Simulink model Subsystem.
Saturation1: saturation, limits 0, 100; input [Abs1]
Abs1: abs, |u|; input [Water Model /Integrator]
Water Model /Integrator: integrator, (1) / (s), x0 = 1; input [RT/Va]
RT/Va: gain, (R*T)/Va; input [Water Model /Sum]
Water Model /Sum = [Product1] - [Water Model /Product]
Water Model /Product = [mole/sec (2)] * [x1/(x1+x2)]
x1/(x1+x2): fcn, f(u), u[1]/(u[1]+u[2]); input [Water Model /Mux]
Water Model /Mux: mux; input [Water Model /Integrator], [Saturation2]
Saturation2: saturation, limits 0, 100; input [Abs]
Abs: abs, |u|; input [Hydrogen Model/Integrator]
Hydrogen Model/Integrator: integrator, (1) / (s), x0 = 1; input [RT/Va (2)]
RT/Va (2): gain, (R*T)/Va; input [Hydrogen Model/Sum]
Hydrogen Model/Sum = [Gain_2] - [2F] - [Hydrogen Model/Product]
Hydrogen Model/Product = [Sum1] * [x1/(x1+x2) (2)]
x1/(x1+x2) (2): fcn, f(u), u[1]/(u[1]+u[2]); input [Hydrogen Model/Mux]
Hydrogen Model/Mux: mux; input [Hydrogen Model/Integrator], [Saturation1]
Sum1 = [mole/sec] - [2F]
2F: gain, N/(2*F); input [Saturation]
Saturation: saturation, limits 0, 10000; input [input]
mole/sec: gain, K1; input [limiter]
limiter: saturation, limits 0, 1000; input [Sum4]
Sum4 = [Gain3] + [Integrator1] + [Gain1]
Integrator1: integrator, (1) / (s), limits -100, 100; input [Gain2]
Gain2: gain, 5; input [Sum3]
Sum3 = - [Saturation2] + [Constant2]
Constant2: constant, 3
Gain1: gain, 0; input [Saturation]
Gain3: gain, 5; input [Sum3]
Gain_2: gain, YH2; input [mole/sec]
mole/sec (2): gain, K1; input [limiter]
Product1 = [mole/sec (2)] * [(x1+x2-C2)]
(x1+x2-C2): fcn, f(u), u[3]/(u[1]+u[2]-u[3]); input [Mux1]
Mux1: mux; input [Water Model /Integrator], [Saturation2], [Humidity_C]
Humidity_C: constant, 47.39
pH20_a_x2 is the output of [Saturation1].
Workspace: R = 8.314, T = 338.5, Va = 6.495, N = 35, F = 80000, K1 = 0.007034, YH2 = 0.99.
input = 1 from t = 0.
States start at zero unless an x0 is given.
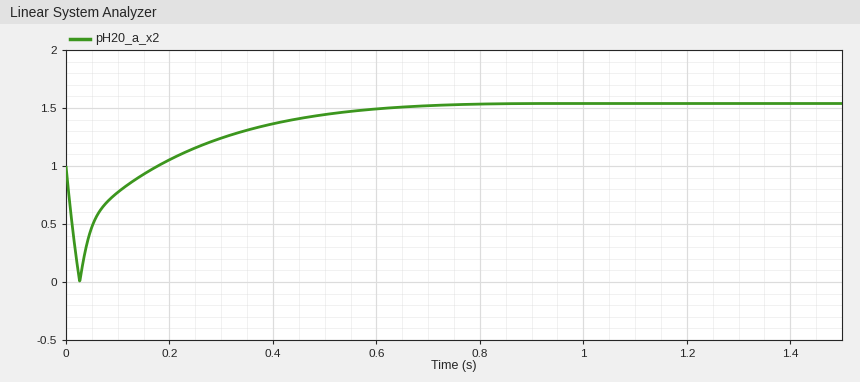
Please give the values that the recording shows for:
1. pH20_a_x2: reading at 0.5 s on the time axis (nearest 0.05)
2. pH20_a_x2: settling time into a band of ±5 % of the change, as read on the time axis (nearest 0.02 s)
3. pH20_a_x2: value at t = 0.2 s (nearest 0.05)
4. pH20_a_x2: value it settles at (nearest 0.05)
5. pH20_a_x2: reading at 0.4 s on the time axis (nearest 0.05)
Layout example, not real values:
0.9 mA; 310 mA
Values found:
1.45; 0.66 s; 1.05; 1.55; 1.35
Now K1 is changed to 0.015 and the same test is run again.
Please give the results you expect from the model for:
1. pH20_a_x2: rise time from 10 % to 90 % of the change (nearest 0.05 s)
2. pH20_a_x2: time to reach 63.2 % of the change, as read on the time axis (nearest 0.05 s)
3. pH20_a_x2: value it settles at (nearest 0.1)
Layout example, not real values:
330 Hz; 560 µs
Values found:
0.20 s; 0.20 s; 1.5
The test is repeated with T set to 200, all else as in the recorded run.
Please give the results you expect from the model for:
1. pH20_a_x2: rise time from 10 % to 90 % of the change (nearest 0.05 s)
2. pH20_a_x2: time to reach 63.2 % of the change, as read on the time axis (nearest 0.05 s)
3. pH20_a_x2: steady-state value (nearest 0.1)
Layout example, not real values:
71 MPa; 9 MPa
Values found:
0.55 s; 0.60 s; 1.6
